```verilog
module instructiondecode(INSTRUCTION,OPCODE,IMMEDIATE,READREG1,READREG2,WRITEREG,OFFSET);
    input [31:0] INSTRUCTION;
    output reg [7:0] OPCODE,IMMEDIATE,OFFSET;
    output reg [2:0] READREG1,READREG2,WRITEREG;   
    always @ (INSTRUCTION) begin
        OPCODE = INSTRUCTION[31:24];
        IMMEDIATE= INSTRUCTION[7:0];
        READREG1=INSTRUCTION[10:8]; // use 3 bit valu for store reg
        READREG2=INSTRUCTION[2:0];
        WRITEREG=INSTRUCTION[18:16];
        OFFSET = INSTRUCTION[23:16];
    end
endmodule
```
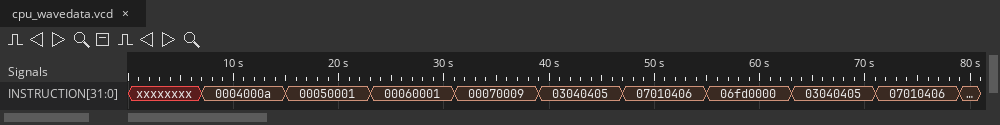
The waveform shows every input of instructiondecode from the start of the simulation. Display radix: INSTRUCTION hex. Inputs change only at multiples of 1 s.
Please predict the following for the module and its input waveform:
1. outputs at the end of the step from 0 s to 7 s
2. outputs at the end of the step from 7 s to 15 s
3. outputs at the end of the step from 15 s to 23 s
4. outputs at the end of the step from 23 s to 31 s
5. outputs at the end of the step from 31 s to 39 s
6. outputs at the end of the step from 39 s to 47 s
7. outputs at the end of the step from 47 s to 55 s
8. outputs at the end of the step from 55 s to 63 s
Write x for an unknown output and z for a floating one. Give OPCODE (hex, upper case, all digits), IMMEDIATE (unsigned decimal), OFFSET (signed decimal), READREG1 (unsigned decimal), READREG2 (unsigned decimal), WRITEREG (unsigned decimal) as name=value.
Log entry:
OPCODE=x, IMMEDIATE=x, OFFSET=x, READREG1=x, READREG2=x, WRITEREG=x
OPCODE=00, IMMEDIATE=10, OFFSET=4, READREG1=0, READREG2=2, WRITEREG=4
OPCODE=00, IMMEDIATE=1, OFFSET=5, READREG1=0, READREG2=1, WRITEREG=5
OPCODE=00, IMMEDIATE=1, OFFSET=6, READREG1=0, READREG2=1, WRITEREG=6
OPCODE=00, IMMEDIATE=9, OFFSET=7, READREG1=0, READREG2=1, WRITEREG=7
OPCODE=03, IMMEDIATE=5, OFFSET=4, READREG1=4, READREG2=5, WRITEREG=4
OPCODE=07, IMMEDIATE=6, OFFSET=1, READREG1=4, READREG2=6, WRITEREG=1
OPCODE=06, IMMEDIATE=0, OFFSET=-3, READREG1=0, READREG2=0, WRITEREG=5
